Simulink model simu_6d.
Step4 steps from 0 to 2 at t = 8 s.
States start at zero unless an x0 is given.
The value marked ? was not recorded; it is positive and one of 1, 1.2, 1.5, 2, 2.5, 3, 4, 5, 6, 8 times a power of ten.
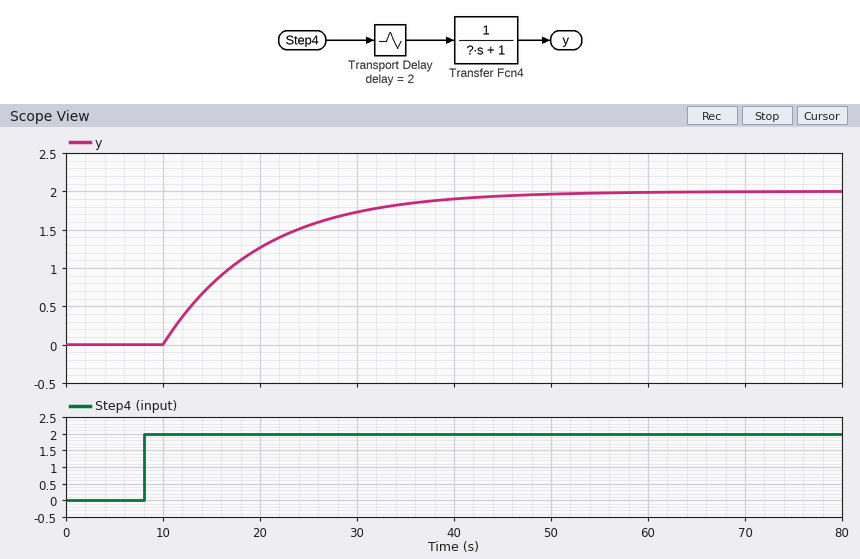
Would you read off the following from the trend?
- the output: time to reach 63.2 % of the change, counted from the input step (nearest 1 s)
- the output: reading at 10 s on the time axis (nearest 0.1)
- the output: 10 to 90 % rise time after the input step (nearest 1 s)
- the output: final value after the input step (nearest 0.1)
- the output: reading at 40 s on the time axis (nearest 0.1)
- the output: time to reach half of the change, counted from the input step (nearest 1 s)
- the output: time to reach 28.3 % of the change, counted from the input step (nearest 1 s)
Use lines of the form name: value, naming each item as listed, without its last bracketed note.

the output: time to reach 63.2 % of the change, counted from the input step: 12 s
the output: reading at 10 s on the time axis: 0.0
the output: 10 to 90 % rise time after the input step: 22 s
the output: final value after the input step: 2.0
the output: reading at 40 s on the time axis: 1.9
the output: time to reach half of the change, counted from the input step: 9 s
the output: time to reach 28.3 % of the change, counted from the input step: 5 s
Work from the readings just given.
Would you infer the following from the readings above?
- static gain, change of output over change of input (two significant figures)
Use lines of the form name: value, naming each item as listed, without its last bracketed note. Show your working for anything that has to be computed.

static gain, change of output over change of input: (2 - 0) / (2 - 0) = 1.0
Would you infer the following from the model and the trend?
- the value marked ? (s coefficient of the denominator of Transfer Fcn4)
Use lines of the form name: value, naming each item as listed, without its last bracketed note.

the value marked ?: 10
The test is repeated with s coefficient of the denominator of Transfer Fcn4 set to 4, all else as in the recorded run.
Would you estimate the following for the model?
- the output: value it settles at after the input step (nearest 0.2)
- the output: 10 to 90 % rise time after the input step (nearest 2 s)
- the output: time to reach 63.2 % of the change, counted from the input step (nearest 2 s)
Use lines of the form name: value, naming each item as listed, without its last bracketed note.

the output: value it settles at after the input step: 2.0
the output: 10 to 90 % rise time after the input step: 8 s
the output: time to reach 63.2 % of the change, counted from the input step: 6 s
